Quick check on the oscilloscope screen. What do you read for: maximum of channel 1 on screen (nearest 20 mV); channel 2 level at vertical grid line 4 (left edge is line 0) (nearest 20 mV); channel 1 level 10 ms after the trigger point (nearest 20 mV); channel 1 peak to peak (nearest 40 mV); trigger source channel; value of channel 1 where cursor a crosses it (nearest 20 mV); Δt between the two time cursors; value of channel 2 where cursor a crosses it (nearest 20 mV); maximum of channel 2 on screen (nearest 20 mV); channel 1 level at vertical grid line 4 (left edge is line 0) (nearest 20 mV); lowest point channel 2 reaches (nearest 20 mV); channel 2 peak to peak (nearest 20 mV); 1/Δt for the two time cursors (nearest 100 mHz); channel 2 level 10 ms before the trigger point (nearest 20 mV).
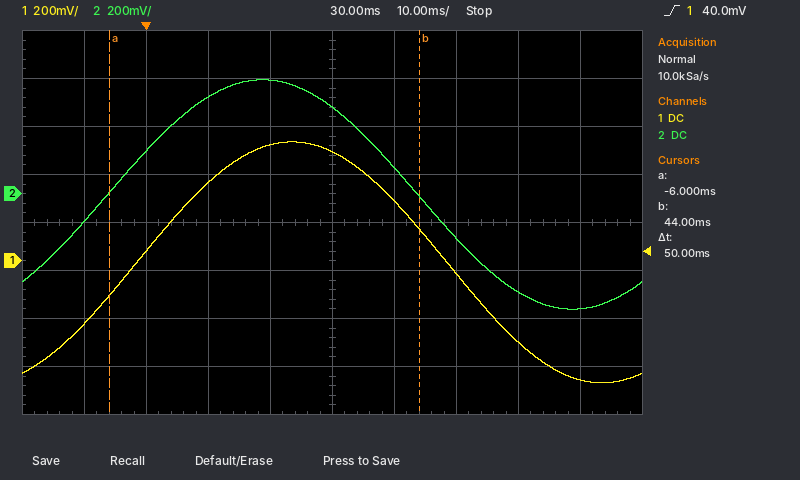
500 mV
480 mV
320 mV
1.00 V
channel 1
-140 mV
50 ms
0 mV
480 mV
480 mV
-480 mV
960 mV
20.0 Hz
-120 mV
